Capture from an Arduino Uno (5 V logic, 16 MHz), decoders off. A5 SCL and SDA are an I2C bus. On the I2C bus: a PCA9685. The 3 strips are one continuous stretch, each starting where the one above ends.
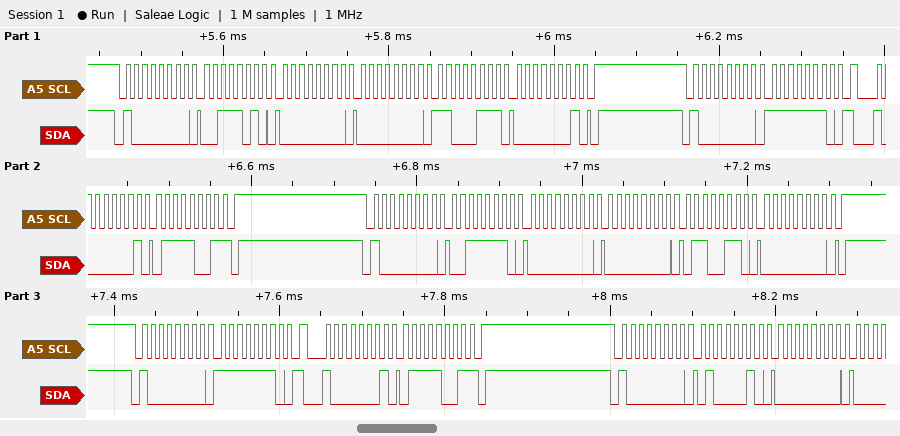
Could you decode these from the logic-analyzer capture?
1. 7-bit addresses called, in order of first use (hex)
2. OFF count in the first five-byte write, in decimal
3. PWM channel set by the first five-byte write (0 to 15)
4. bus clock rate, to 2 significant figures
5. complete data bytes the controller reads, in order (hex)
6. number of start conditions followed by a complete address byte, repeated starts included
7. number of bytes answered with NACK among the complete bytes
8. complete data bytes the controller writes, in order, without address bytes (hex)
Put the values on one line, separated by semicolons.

0x40; 455; 13; 100 kHz; 79 79; 7; 2; 3A 00 00 C7 01 FE 3E 00 00 66 00 FE 42 00
